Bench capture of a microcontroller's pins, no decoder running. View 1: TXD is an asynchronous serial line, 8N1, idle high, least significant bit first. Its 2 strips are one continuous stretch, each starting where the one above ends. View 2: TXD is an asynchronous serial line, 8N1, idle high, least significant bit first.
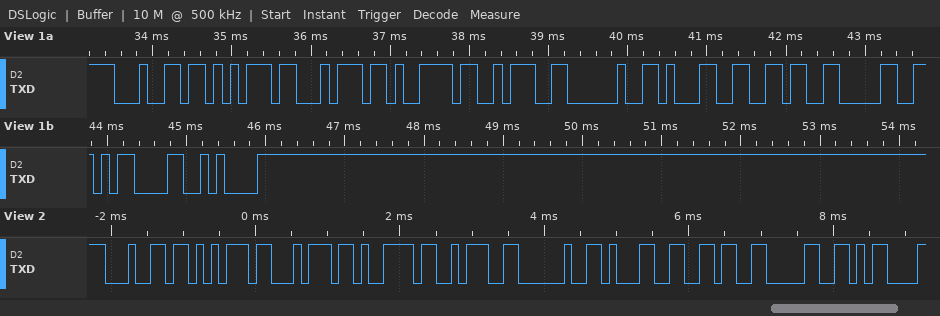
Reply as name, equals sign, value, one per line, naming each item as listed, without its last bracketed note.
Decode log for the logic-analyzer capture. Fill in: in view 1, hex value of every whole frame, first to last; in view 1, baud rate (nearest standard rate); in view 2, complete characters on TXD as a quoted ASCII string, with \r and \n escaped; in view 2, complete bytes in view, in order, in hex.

in view 1, hex value of every whole frame, first to last = 0x64 0x75 0x74 0x79 0x3A 0x20 0x31 0x36 0x30 0x0D 0x0A
in view 1, baud rate = 9600 baud
in view 2, complete characters on TXD as a quoted ASCII string, with \r and \n escaped = "duty: 160\r"
in view 2, complete bytes in view, in order, in hex = 0x64 0x75 0x74 0x79 0x3A 0x20 0x31 0x36 0x30 0x0D
